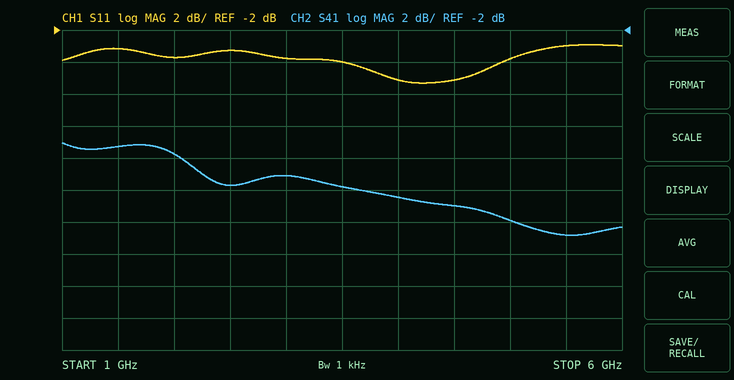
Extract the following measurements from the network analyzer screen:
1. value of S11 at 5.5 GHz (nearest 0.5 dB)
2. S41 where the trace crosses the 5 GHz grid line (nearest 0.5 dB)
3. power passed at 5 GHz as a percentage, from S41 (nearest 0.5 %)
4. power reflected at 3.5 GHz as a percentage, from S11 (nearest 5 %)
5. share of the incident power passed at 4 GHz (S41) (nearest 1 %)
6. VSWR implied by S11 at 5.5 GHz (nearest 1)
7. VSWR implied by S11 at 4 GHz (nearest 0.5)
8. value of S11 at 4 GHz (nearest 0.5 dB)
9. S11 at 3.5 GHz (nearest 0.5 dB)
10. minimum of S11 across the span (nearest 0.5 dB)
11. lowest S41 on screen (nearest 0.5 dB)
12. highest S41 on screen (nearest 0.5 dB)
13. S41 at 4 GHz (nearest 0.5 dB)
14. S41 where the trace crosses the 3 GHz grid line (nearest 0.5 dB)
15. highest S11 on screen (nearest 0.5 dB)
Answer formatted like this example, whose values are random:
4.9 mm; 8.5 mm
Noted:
-3.0 dB; -14.0 dB; 4.0 %; 40 %; 6 %; 6; 3.5; -5.0 dB; -4.0 dB; -5.5 dB; -15.0 dB; -9.0 dB; -12.5 dB; -11.0 dB; -3.0 dB
